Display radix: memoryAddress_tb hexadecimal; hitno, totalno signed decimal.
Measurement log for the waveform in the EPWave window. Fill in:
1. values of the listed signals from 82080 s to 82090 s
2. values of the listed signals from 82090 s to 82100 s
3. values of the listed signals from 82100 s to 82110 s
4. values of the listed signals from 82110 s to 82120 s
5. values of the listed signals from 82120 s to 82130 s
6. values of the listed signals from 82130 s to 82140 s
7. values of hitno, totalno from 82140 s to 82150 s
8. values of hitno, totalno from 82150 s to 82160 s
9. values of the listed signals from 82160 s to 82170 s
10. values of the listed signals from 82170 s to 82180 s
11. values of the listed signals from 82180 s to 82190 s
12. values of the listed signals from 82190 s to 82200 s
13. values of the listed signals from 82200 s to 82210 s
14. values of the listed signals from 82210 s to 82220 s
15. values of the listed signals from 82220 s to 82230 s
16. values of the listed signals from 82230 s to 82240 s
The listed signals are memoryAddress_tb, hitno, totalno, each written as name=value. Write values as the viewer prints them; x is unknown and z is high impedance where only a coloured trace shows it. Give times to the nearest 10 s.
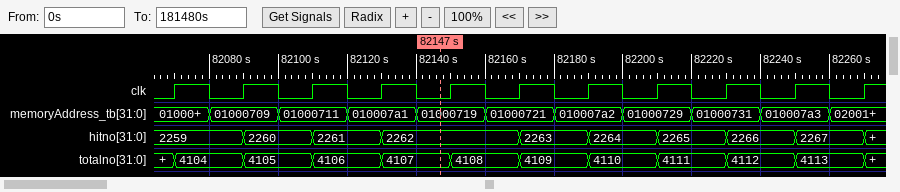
memoryAddress_tb=01000709, hitno=2259, totalno=4104
memoryAddress_tb=01000709, hitno=2260, totalno=4105
memoryAddress_tb=01000711, hitno=2260, totalno=4105
memoryAddress_tb=01000711, hitno=2261, totalno=4106
memoryAddress_tb=010007a1, hitno=2261, totalno=4106
memoryAddress_tb=010007a1, hitno=2262, totalno=4107
hitno=2262, totalno=4107
hitno=2262, totalno=4108
memoryAddress_tb=01000721, hitno=2262, totalno=4108
memoryAddress_tb=01000721, hitno=2263, totalno=4109
memoryAddress_tb=010007a2, hitno=2263, totalno=4109
memoryAddress_tb=010007a2, hitno=2264, totalno=4110
memoryAddress_tb=01000729, hitno=2264, totalno=4110
memoryAddress_tb=01000729, hitno=2265, totalno=4111
memoryAddress_tb=01000731, hitno=2265, totalno=4111
memoryAddress_tb=01000731, hitno=2266, totalno=4112
